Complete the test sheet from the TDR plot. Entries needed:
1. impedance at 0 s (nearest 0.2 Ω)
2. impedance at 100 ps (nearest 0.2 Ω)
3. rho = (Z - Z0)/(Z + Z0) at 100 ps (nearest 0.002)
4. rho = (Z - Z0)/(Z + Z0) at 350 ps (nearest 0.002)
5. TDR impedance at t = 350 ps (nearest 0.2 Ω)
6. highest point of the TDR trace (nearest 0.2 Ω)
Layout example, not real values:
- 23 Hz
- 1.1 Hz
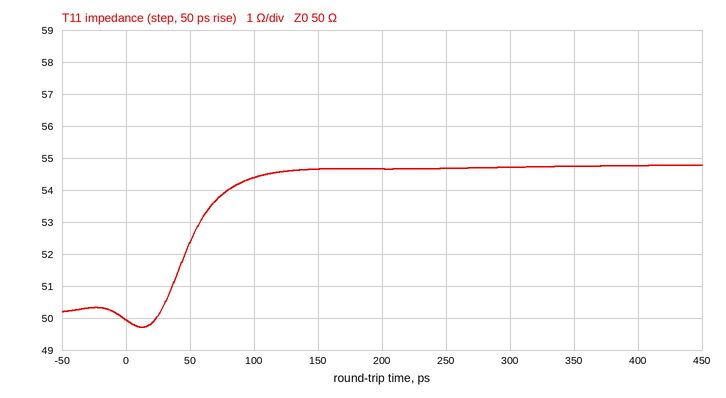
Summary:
- 50.0 Ω
- 54.4 Ω
- +0.042
- +0.046
- 54.8 Ω
- 54.8 Ω
